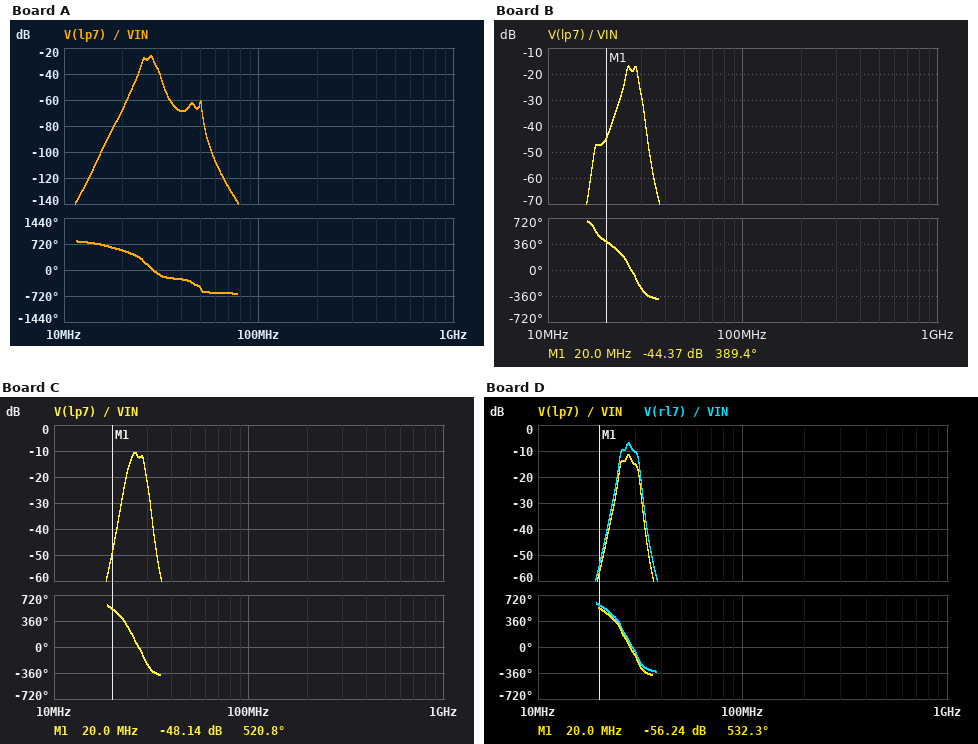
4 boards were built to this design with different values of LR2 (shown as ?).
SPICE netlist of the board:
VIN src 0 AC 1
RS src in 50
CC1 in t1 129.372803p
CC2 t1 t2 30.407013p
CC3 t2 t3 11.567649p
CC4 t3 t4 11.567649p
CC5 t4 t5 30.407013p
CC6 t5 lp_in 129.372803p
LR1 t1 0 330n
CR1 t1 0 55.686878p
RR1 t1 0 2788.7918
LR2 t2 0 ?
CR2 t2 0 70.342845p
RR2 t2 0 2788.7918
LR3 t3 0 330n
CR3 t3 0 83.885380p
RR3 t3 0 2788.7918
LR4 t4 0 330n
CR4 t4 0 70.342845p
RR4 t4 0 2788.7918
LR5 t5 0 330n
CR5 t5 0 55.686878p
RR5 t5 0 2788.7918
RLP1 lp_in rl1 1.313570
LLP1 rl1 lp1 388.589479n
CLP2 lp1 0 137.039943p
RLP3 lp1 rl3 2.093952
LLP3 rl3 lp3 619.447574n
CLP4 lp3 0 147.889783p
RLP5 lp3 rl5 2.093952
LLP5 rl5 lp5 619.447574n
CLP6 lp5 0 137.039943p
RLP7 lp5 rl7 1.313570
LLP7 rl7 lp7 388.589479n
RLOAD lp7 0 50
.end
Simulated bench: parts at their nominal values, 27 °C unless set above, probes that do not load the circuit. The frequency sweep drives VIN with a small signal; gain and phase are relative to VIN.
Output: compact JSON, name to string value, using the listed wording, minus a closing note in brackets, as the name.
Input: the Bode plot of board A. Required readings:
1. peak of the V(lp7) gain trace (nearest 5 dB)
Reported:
{"peak of the V(lp7) gain trace": "-25 dB"}
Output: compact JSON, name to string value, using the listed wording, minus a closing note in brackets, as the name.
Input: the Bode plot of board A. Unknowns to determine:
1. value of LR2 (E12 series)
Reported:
{"value of LR2": "120 nH"}
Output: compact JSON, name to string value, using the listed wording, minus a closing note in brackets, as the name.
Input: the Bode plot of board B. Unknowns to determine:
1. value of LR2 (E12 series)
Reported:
{"value of LR2": "680 nH"}
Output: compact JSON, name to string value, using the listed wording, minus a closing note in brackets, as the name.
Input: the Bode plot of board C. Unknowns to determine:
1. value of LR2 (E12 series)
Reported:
{"value of LR2": "390 nH"}
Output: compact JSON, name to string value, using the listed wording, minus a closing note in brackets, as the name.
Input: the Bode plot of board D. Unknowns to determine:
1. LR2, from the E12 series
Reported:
{"LR2, from the E12 series": "270 nH"}
